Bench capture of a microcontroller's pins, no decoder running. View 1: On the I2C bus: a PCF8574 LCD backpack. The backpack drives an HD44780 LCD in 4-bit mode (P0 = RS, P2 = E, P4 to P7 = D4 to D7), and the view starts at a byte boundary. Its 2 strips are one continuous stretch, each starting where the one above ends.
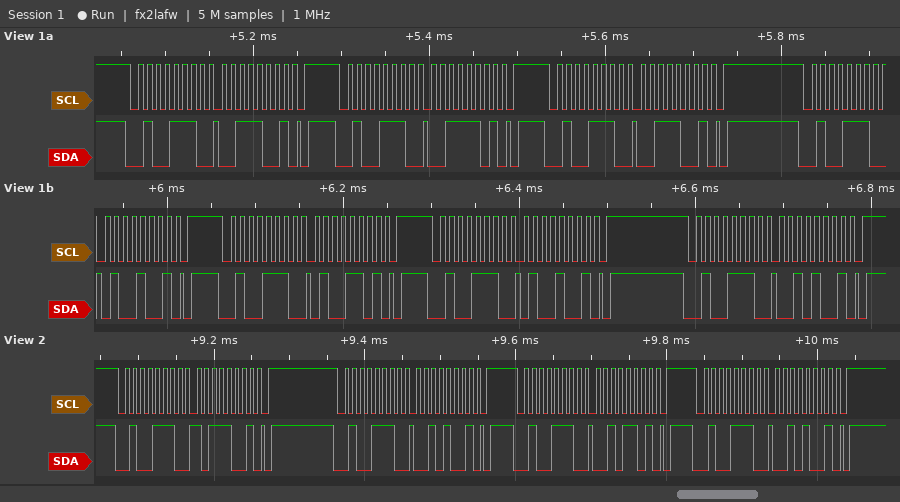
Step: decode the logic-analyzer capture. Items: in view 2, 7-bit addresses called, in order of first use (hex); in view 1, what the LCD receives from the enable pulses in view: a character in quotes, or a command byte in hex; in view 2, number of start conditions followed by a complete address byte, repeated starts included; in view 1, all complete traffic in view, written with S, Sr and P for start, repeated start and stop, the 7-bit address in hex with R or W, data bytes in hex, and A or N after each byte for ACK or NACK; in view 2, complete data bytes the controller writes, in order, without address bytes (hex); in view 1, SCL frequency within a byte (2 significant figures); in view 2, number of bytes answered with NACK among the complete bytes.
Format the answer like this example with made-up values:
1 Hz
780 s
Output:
0x27
'4'
4
S 27W A 39 A P S 27W A 3D A P S 27W A 39 A P S 27W A 49 A P S 27W A 4D A P S 27W A 49 A P S 27W A 29 A P
B9 29 2D 29
100 kHz
0
